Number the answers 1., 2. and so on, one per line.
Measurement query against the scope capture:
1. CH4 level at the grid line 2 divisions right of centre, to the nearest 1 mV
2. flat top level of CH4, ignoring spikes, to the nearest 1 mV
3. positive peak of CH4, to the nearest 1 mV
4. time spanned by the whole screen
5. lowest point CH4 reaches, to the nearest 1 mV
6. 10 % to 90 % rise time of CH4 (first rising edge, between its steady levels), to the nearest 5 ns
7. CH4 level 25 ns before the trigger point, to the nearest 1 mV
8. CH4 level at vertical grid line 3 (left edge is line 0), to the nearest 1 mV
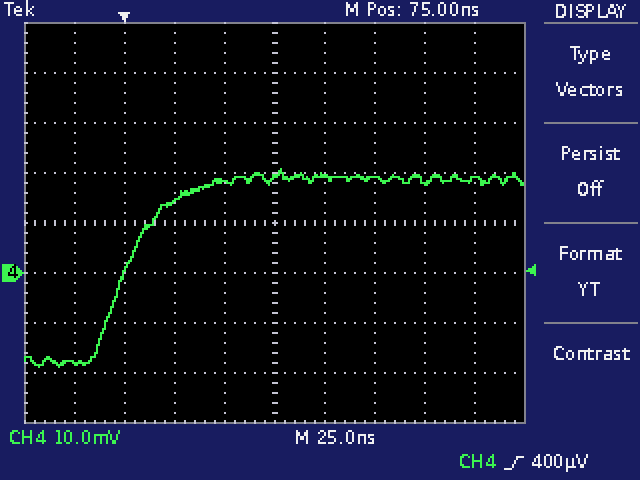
1. 19 mV
2. 19 mV
3. 21 mV
4. 250 ns
5. -19 mV
6. 40 ns
7. -18 mV
8. 14 mV
